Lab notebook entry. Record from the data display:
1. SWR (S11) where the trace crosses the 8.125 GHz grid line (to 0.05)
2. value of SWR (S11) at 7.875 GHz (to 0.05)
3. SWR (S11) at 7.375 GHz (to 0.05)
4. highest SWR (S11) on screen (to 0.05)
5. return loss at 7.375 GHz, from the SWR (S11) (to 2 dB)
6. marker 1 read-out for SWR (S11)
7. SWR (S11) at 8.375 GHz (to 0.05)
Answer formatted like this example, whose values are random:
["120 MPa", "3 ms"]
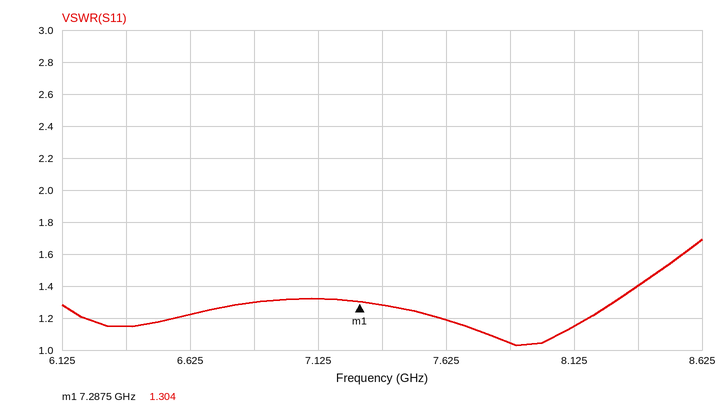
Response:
["1.15", "1.05", "1.30", "1.70", "18 dB", "1.304", "1.40"]
